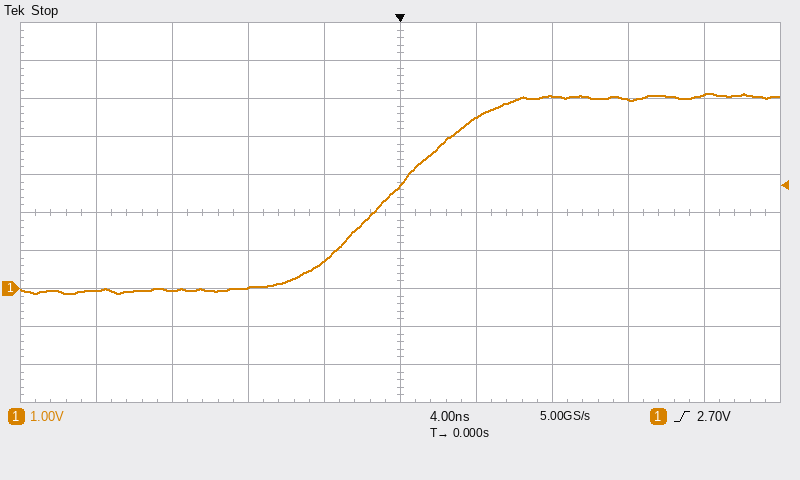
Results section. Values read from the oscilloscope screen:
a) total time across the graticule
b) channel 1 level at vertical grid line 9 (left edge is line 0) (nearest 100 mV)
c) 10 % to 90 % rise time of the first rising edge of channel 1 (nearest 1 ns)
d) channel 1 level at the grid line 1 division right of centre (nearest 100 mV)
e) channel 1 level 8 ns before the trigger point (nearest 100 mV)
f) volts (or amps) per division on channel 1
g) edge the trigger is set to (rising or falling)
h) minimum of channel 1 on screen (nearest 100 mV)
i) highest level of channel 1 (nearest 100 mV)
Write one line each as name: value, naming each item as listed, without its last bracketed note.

total time across the graticule: 40 ns
channel 1 level at vertical grid line 9 (left edge is line 0): 5.1 V
10 % to 90 % rise time of the first rising edge of channel 1: 9 ns
channel 1 level at the grid line 1 division right of centre: 4.5 V
channel 1 level 8 ns before the trigger point: 0.0 V
volts (or amps) per division on channel 1: 1 V
edge the trigger is set to: rising
minimum of channel 1 on screen: -100 mV
highest level of channel 1: 5.1 V
